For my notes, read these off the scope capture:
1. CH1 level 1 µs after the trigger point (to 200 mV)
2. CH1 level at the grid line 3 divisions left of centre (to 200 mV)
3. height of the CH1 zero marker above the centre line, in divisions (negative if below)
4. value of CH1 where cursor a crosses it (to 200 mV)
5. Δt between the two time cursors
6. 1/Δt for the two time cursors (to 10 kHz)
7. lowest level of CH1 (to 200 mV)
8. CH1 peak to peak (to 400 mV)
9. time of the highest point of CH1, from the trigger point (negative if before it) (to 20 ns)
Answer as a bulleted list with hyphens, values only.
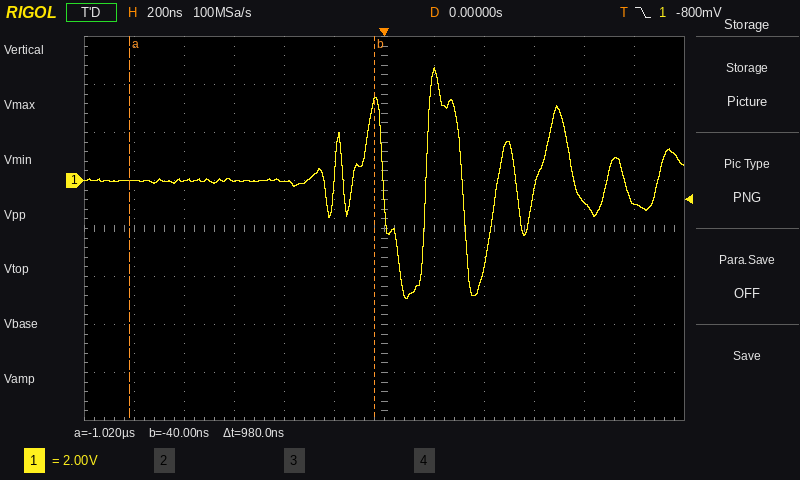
- -1.0 V
- 0.0 V
- +1.0 div
- 0.0 V
- 980 ns
- 1.02 MHz
- -5.0 V
- 9.6 V
- +200 ns
